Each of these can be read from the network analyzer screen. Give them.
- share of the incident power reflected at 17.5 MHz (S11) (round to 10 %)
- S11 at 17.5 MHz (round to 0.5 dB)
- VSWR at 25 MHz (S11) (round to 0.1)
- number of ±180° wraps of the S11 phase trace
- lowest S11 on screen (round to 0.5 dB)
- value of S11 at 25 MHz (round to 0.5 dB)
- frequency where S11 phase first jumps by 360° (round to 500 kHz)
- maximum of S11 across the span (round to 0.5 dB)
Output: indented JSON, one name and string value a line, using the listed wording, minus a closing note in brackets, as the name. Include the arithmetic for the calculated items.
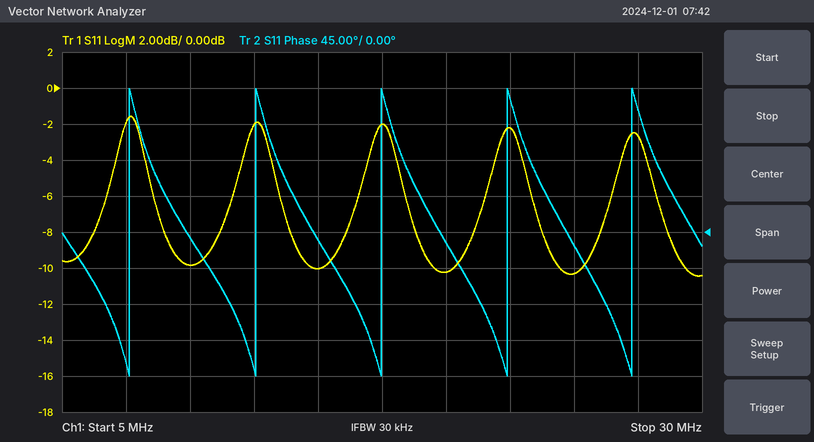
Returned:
{
  "share of the incident power reflected at 17.5 MHz (S11)": "10^(-2/10) ≈ 63.1 %, so 60 % to the nearest 10 %",
  "S11 at 17.5 MHz": "-2.0 dB",
  "VSWR at 25 MHz (S11)": "|Γ| = 10^(-10.5/20) = 0.2985; VSWR = (1 + 0.2985)/(1 − 0.2985) ≈ 1.9",
  "number of ±180° wraps of the S11 phase trace": "5",
  "lowest S11 on screen": "-10.5 dB",
  "value of S11 at 25 MHz": "-10.5 dB",
  "frequency where S11 phase first jumps by 360°": "7.5 MHz",
  "maximum of S11 across the span": "-1.5 dB"
}
